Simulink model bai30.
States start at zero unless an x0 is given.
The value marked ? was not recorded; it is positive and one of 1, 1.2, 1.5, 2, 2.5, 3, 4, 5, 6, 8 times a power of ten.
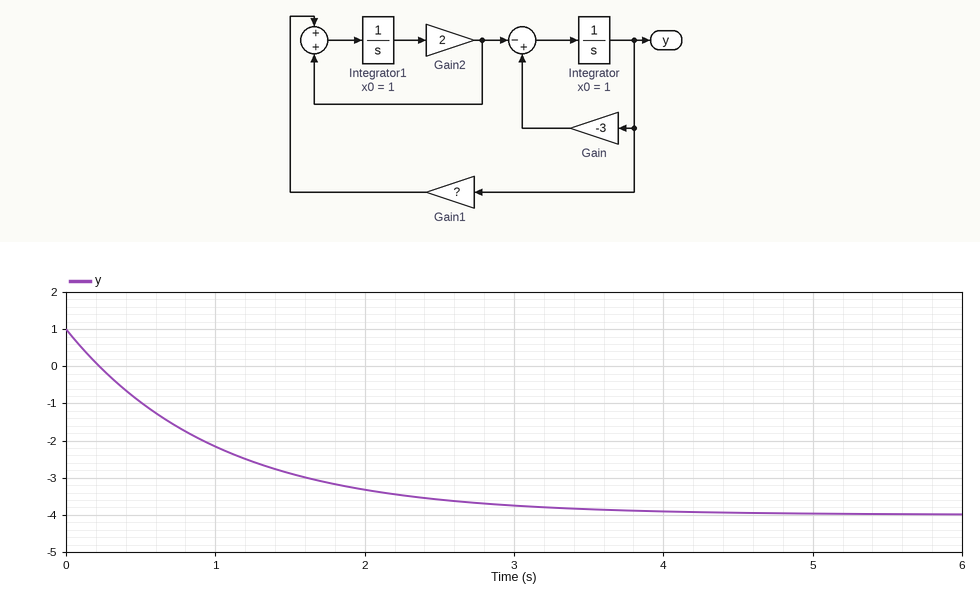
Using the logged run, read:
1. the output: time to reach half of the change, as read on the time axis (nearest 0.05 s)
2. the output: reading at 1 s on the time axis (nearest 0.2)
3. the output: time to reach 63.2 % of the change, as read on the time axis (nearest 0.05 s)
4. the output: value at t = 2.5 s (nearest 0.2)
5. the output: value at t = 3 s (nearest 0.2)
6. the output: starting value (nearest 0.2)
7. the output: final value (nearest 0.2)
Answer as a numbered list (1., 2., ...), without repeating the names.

1. 0.70 s
2. -2.2
3. 1.00 s
4. -3.6
5. -3.8
6. 1.0
7. -4.0
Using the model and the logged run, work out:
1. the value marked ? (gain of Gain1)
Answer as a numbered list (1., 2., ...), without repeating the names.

1. 3
